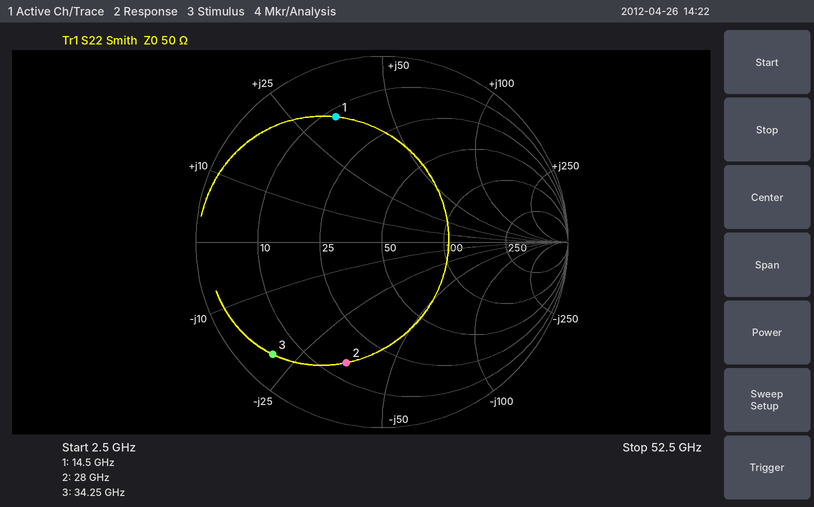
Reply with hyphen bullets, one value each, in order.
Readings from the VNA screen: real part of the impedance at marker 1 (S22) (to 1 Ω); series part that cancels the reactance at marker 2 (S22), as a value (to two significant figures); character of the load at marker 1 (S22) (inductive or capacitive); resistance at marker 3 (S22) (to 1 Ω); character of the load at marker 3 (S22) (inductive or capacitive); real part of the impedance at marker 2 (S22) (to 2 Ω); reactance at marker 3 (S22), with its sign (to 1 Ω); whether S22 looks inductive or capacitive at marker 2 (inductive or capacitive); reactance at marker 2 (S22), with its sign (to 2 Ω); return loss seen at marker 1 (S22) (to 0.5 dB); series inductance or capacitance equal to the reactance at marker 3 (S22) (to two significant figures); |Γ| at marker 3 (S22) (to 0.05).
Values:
- 12 Ω
- 200 pH
- inductive
- 5 Ω
- capacitive
- 14 Ω
- -21 Ω
- capacitive
- -36 Ω
- 3.0 dB
- 220 fF
- 0.85
